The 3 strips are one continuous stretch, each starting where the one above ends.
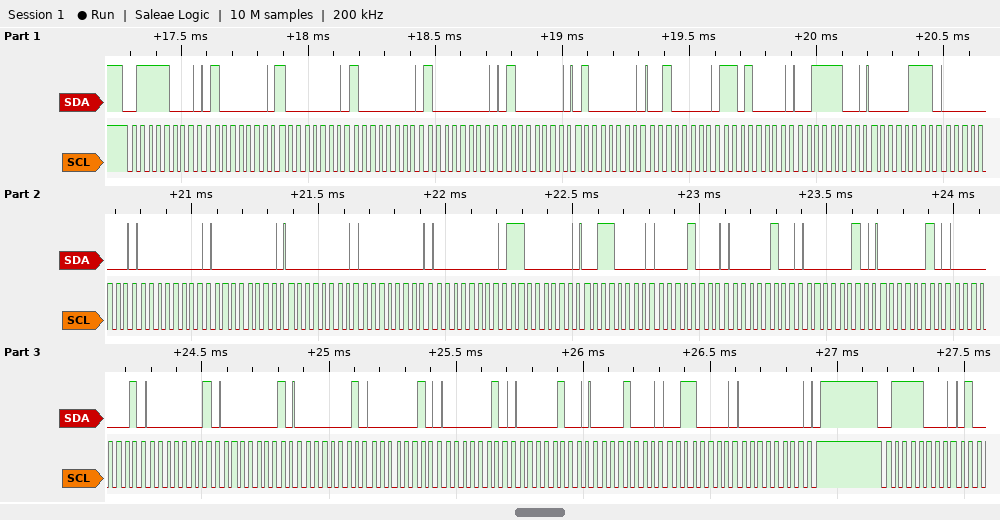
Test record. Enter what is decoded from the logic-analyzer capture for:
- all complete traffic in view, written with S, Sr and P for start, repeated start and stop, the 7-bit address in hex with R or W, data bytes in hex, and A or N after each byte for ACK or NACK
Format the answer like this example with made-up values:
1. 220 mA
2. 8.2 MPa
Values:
1. S 3CW A 40 A 80 A 80 A 80 A 40 A 40 A 20 A D0 A 3C A 07 A 00 A 00 A 00 A 00 A 00 A 00 A C0 A 30 A 08 A 04 A 02 A 02 A 01 A 01 A 01 A 01 A 02 A 02 A 04 A 08 A 30 A 00 A P S 3CW A
